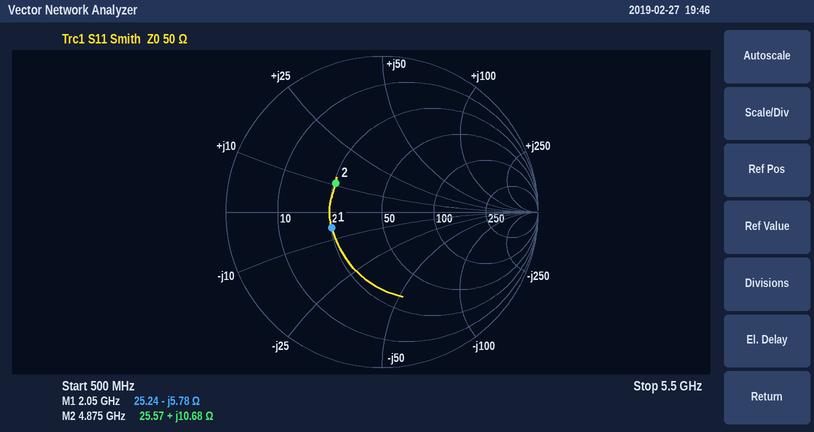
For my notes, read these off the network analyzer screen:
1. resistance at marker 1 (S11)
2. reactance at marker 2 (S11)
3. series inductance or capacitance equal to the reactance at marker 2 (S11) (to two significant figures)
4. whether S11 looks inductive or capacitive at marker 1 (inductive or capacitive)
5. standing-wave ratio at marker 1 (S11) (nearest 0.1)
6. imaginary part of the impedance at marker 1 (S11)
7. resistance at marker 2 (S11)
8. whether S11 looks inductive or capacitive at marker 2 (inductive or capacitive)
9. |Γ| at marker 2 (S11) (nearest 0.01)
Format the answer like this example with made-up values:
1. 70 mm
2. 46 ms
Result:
1. 25.24 Ω
2. +10.68 Ω
3. 350 pH
4. capacitive
5. 2.0
6. -5.78 Ω
7. 25.57 Ω
8. inductive
9. 0.35
